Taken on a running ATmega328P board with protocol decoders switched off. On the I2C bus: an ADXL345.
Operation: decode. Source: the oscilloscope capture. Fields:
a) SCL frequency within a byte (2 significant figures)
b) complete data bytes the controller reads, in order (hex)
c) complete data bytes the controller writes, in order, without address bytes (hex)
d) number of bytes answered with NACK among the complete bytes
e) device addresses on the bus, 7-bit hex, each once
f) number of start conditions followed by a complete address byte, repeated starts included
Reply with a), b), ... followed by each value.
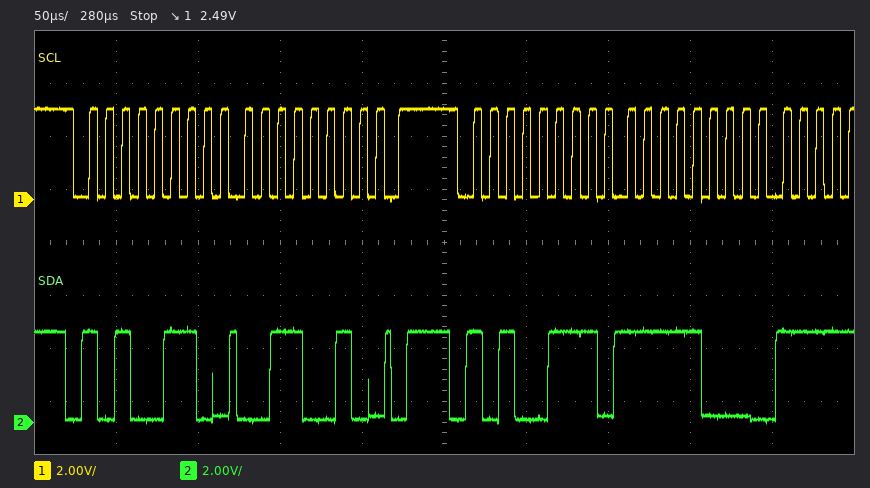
a) 100 kHz
b) F8
c) 32
d) 0
e) 0x53
f) 2
